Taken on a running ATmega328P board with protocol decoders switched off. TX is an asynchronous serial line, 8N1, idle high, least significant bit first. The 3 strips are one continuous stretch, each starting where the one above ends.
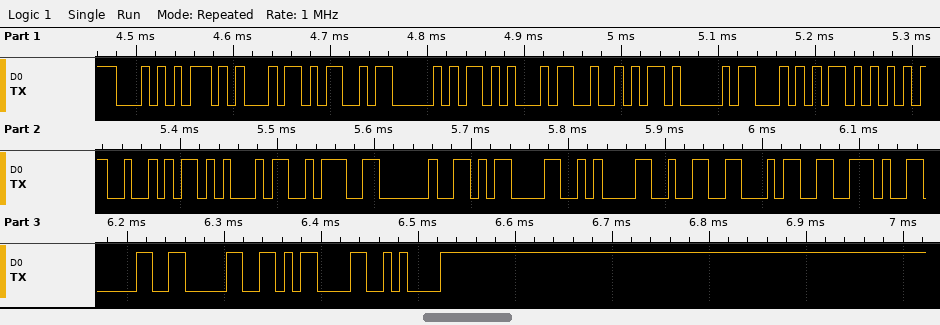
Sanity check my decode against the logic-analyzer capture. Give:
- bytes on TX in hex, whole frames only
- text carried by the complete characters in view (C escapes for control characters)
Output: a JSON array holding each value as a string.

["0x54 0x45 0x4D 0x50 0x45 0x52 0x41 0x54 0x55 0x52 0x45 0x3A 0x20 0x0D 0x0A 0x32 0x34 0x2E 0x30 0x30 0x0D 0x0A", "\"TEMPERATURE: \\r\\n24.00\\r\\n\""]
